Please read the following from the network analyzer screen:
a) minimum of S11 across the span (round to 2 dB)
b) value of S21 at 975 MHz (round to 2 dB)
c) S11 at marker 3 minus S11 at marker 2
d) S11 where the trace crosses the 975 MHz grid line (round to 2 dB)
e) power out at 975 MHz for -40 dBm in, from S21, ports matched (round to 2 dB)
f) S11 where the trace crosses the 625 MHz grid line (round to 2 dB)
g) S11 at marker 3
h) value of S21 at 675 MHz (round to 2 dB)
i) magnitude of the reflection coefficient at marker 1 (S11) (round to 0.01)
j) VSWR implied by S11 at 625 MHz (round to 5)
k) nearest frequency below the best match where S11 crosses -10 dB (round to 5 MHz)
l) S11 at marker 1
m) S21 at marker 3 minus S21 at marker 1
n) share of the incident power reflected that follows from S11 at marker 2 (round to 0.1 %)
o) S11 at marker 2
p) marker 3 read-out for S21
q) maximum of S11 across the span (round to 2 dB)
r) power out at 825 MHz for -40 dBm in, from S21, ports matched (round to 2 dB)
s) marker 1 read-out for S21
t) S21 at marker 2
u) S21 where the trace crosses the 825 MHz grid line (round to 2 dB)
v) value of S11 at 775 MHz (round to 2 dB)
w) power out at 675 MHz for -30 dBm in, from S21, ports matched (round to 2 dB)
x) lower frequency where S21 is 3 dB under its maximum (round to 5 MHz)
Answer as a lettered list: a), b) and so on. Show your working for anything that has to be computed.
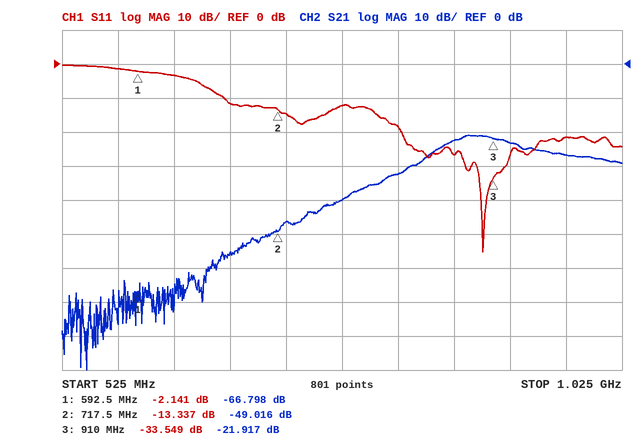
a) -56 dB
b) -26 dB
c) -33.549 − (-13.337) = -20.212 dB
d) -22 dB
e) -40 dBm + (-26 dB) = -66 dBm
f) -4 dB
g) -33.549 dB
h) -56 dB
i) 10^(-2.141/20) ≈ 0.78
j) |Γ| = 10^(-4/20) = 0.6310; VSWR = (1 + 0.6310)/(1 − 0.6310) ≈ 4.42, so 5 to the nearest 5
k) 670 MHz
l) -2.141 dB
m) -21.917 − (-66.798) = 44.881 dB
n) 10^(-13.337/10) ≈ 4.6 %
o) -13.337 dB
p) -21.917 dB
q) 0 dB
r) -40 dBm + (-32 dB) = -72 dBm
s) -66.798 dB
t) -49.016 dB
u) -32 dB
v) -12 dB
w) -30 dBm + (-56 dB) = -86 dBm
x) 865 MHz
